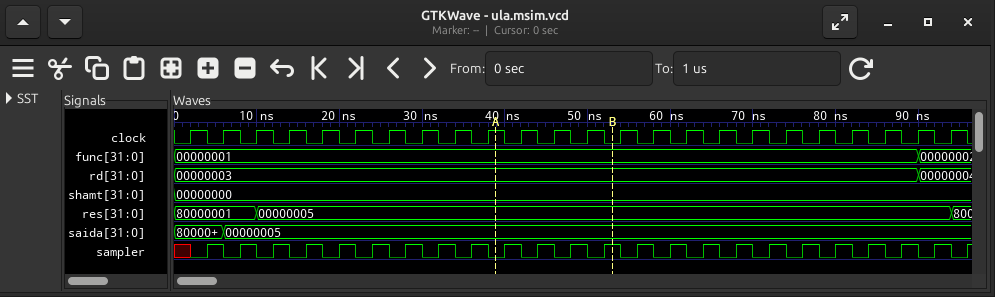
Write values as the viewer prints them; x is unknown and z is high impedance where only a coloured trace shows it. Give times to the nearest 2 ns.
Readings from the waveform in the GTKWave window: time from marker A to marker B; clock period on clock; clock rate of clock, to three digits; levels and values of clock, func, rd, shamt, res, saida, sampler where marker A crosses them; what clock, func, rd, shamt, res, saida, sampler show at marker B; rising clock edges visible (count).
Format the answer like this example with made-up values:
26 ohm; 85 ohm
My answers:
14 ns; 4 ns; 250 MHz; clock=1, func=00000001, rd=00000003, shamt=00000000, res=00000005, saida=00000005, sampler=0; clock=0, func=00000001, rd=00000003, shamt=00000000, res=00000005, saida=00000005, sampler=1; 24
